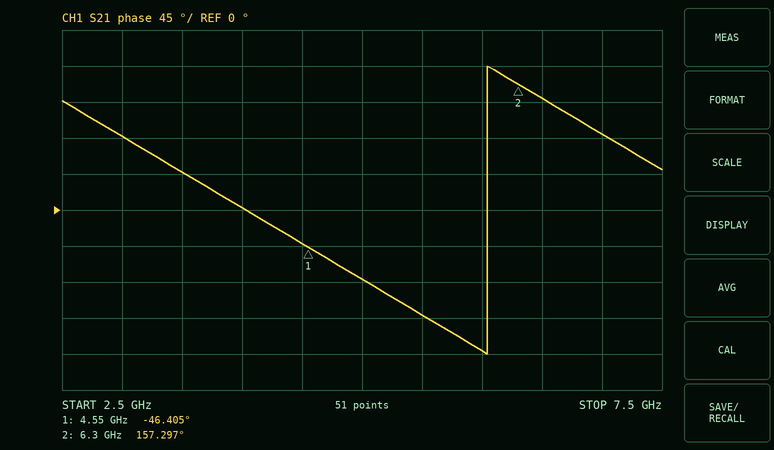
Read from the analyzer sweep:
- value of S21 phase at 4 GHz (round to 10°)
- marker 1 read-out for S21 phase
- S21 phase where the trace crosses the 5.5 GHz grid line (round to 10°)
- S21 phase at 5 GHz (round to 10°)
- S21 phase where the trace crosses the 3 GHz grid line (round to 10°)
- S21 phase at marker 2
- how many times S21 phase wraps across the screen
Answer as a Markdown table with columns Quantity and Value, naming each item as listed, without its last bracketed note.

| Quantity | Value |
|---|---|
| value of S21 phase at 4 GHz | 0° |
| marker 1 read-out for S21 phase | -46.405° |
| S21 phase where the trace crosses the 5.5 GHz grid line | -130° |
| S21 phase at 5 GHz | -90° |
| S21 phase where the trace crosses the 3 GHz grid line | 90° |
| S21 phase at marker 2 | 157.297° |
| how many times S21 phase wraps across the screen | 1 |
